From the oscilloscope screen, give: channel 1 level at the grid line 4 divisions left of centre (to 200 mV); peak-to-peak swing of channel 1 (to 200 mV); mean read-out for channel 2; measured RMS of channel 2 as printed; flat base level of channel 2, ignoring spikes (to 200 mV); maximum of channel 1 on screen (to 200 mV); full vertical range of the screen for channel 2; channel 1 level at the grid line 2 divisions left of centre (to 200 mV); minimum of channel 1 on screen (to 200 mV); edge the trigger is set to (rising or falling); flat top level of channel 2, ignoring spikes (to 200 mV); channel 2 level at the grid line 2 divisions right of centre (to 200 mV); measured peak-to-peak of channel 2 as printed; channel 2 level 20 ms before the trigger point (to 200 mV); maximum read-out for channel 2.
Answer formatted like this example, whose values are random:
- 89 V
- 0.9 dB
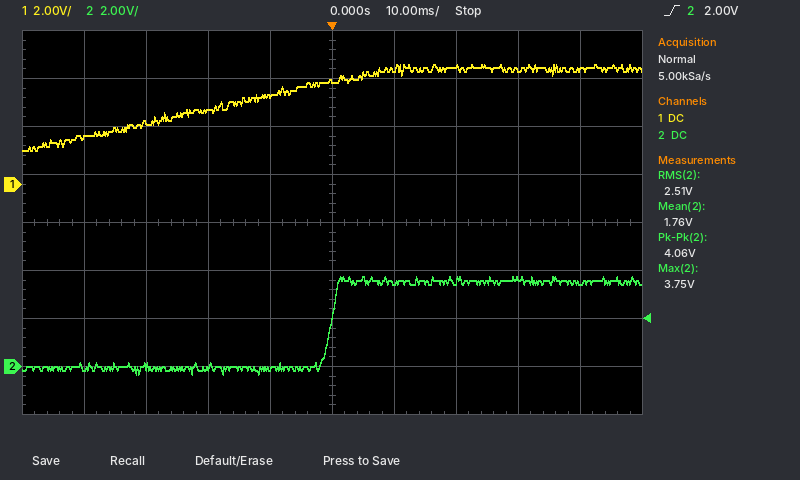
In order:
- 2.0 V
- 3.6 V
- 1.76 V
- 2.51 V
- 0.0 V
- 5.0 V
- 16 V
- 3.0 V
- 1.4 V
- rising
- 3.6 V
- 3.6 V
- 4.06 V
- 0.0 V
- 3.75 V
